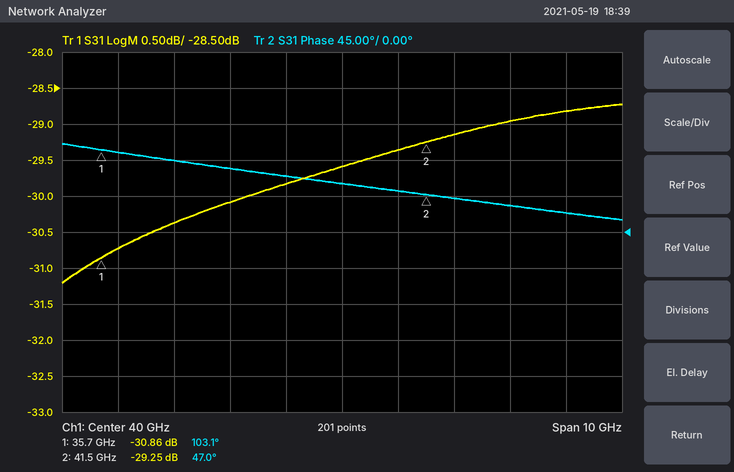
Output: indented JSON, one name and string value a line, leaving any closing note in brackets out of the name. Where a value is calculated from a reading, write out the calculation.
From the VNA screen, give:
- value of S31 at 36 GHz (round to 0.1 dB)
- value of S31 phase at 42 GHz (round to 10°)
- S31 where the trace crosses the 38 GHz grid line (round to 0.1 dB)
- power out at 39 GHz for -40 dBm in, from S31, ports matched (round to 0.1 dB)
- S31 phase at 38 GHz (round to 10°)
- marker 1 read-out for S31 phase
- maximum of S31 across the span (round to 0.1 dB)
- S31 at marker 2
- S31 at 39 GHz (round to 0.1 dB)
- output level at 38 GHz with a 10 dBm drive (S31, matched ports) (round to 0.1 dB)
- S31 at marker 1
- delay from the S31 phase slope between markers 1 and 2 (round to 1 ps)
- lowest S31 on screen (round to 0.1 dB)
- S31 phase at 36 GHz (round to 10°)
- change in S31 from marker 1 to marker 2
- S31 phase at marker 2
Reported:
{
  "value of S31 at 36 GHz": "-30.7 dB",
  "value of S31 phase at 42 GHz": "40°",
  "S31 where the trace crosses the 38 GHz grid line": "-30.1 dB",
  "power out at 39 GHz for -40 dBm in, from S31, ports matched": "-40 dBm + (-29.8 dB) = -69.8 dBm",
  "S31 phase at 38 GHz": "80°",
  "marker 1 read-out for S31 phase": "103.1°",
  "maximum of S31 across the span": "-28.7 dB",
  "S31 at marker 2": "-29.25 dB",
  "S31 at 39 GHz": "-29.8 dB",
  "output level at 38 GHz with a 10 dBm drive (S31, matched ports)": "10 dBm + (-30.1 dB) = -20.1 dBm",
  "S31 at marker 1": "-30.86 dB",
  "delay from the S31 phase slope between markers 1 and 2": "−(47° − (103.1°))/(360° × 5.8 GHz) ≈ 27 ps",
  "lowest S31 on screen": "-31.2 dB",
  "S31 phase at 36 GHz": "100°",
  "change in S31 from marker 1 to marker 2": "-29.25 − (-30.86) = 1.61 dB",
  "S31 phase at marker 2": "47.0°"
}
